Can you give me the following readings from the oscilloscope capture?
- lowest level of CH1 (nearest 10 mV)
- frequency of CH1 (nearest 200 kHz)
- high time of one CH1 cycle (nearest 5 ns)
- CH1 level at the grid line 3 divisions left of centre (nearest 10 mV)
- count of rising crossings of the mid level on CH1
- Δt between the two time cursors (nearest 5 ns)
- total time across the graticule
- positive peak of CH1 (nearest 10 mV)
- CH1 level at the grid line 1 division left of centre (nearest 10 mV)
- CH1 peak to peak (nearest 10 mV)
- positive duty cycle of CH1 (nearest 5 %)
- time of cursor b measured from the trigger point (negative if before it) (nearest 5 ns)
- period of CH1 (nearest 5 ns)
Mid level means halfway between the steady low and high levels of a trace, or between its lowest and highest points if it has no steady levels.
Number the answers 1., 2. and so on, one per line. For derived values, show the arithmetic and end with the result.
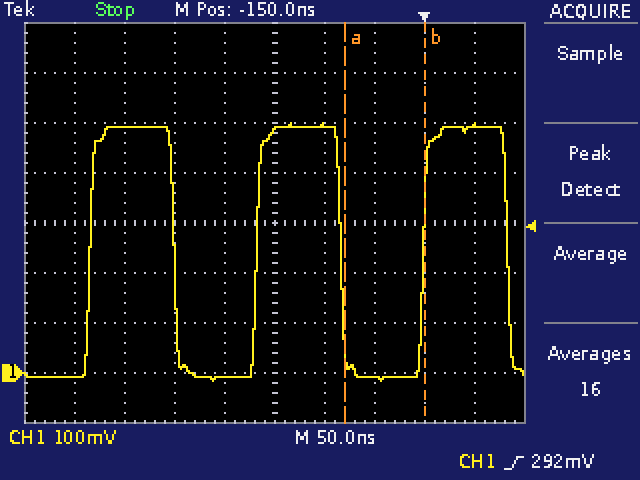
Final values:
1. -20 mV
2. 1 / 165 ns ≈ 6.06 MHz, so 6.0 MHz to the nearest 200 kHz
3. 85 ns
4. 490 mV
5. 3
6. 80 ns
7. 500 ns
8. 500 mV
9. -10 mV
10. 500 mV − (-20 mV) = 520 mV
11. 85 ns / 165 ns ≈ 51.5 %, so 50 % to the nearest 5 %
12. 0 ns
13. 165 ns
